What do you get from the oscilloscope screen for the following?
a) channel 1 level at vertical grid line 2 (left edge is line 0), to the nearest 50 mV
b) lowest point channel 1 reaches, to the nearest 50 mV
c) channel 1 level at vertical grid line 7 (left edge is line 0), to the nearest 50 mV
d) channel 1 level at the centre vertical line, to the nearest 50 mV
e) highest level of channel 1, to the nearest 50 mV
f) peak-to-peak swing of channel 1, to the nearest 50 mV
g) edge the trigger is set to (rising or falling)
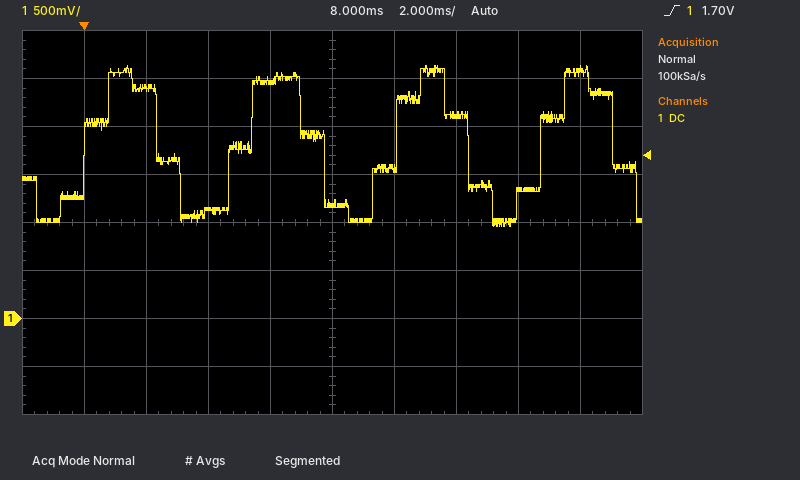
2.40 V
950 mV
2.10 V
1.20 V
2.65 V
1.70 V
rising
